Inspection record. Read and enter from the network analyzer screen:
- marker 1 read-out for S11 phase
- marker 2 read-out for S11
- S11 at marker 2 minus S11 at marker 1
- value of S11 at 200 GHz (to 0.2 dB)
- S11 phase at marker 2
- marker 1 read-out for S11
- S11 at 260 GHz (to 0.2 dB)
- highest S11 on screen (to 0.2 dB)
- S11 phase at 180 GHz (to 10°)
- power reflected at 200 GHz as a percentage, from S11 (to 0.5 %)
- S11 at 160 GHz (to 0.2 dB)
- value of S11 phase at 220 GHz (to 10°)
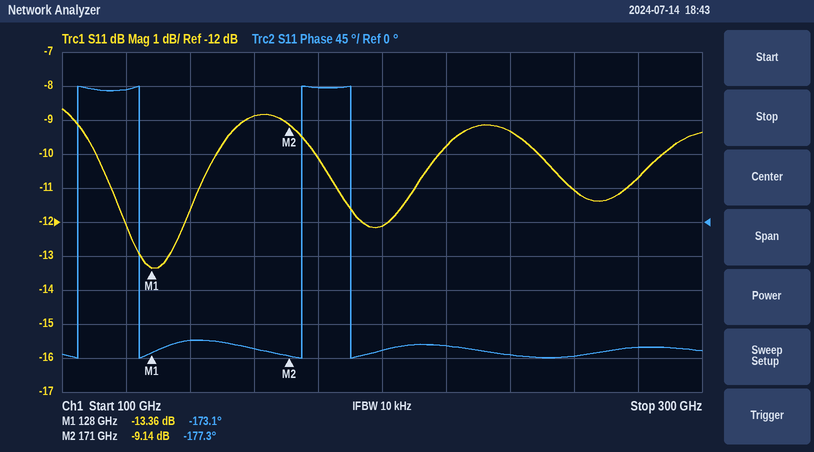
-173.1°
-9.14 dB
4.22 dB
-12.2 dB
-177.3°
-13.36 dB
-11.0 dB
-8.6 dB
180°
6.0 %
-8.8 dB
-160°
